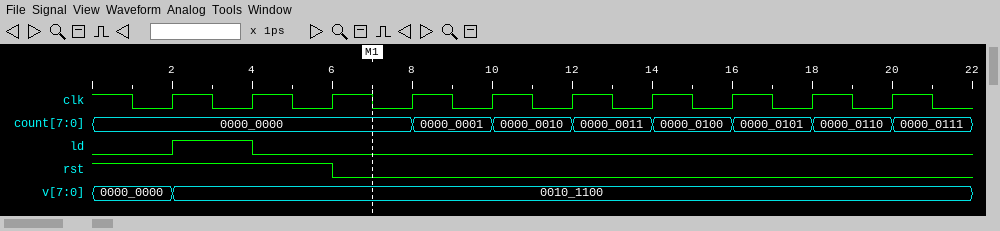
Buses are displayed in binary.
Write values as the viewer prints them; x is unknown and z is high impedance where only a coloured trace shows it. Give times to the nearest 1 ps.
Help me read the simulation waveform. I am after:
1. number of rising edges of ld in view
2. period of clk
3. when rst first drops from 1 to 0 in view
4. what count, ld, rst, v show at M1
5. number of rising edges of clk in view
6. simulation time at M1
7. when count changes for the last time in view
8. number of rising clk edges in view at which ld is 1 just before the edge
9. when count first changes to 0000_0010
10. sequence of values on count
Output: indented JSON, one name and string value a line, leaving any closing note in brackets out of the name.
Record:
{
  "number of rising edges of ld in view": "1",
  "period of clk": "2 ps",
  "when rst first drops from 1 to 0 in view": "6 ps",
  "what count, ld, rst, v show at M1": "count=0000_0000, ld=0, rst=0, v=0010_1100",
  "number of rising edges of clk in view": "10",
  "simulation time at M1": "7 ps",
  "when count changes for the last time in view": "20 ps",
  "number of rising clk edges in view at which ld is 1 just before the edge": "1",
  "when count first changes to 0000_0010": "10 ps",
  "sequence of values on count": "0000_0000, 0000_0001, 0000_0010, 0000_0011, 0000_0100, 0000_0101, 0000_0110, 0000_0111"
}
